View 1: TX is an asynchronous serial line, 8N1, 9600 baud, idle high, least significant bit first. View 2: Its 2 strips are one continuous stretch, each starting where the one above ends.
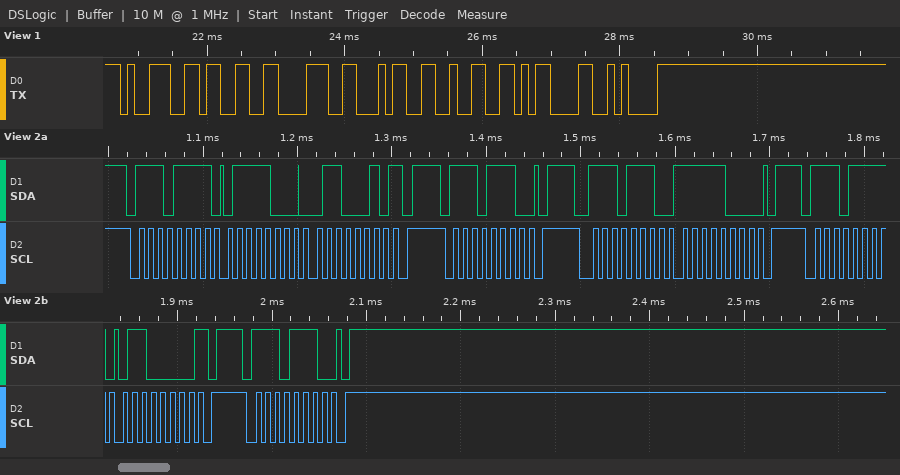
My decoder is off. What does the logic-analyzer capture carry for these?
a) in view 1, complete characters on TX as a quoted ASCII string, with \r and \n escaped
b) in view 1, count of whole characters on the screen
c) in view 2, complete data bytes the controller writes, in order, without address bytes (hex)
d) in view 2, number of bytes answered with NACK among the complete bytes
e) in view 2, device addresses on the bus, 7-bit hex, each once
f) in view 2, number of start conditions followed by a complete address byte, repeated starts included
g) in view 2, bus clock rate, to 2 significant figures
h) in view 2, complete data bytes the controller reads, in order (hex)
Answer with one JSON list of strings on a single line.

["\"93842\\r\\n\"", "7", "F8", "2", "0x77", "5", "100 kHz", "78 62 60"]
